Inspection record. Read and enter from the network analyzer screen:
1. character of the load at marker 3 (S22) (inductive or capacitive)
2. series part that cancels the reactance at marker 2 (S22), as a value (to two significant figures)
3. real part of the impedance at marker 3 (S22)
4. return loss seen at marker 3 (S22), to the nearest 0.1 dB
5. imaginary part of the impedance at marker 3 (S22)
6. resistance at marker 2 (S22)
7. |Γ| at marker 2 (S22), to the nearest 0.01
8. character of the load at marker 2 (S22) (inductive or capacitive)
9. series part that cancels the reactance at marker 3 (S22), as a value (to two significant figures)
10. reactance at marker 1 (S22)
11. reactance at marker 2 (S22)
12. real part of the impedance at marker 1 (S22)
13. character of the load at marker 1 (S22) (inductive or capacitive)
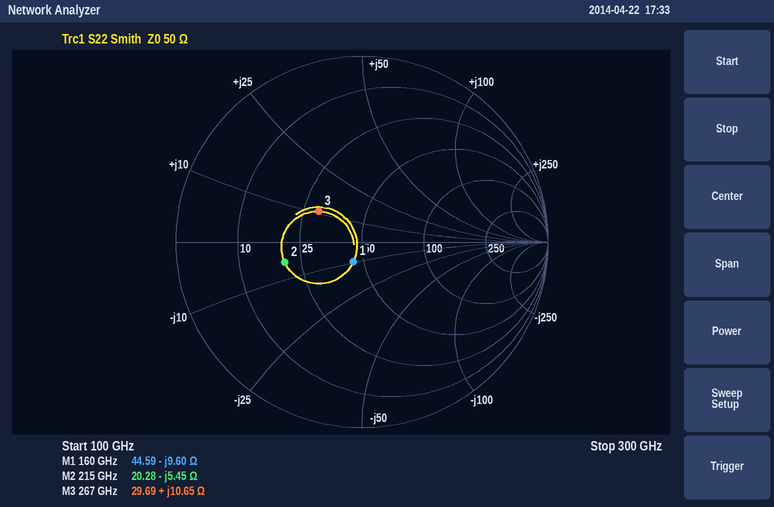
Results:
inductive
4.0 pH
29.69 Ω
10.9 dB
+10.65 Ω
20.28 Ω
0.43
capacitive
56 fF
-9.60 Ω
-5.45 Ω
44.59 Ω
capacitive
